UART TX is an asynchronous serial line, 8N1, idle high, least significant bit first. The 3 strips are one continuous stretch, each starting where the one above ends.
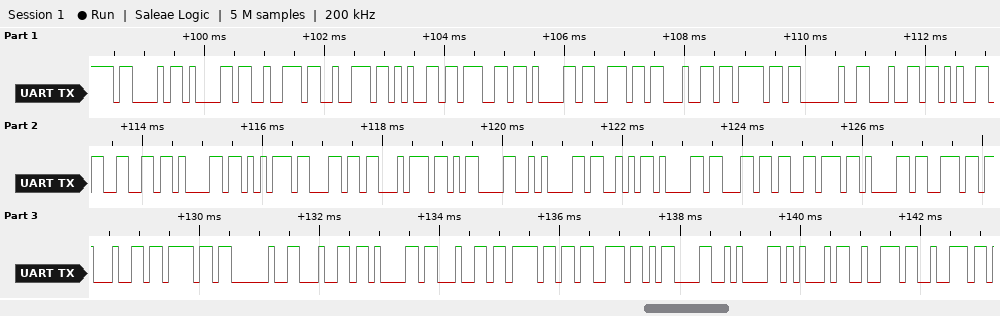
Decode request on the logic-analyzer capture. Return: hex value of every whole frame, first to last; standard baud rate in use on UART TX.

43 61 72 72 65 67 61 6E 64 6F 20 64 65 66 61 75 6C 74 0D 0A 53 61 6C 76 61 6E 64 6F 20 64 61 64 6F 73 0D 0A 45 72 72
9600 baud
